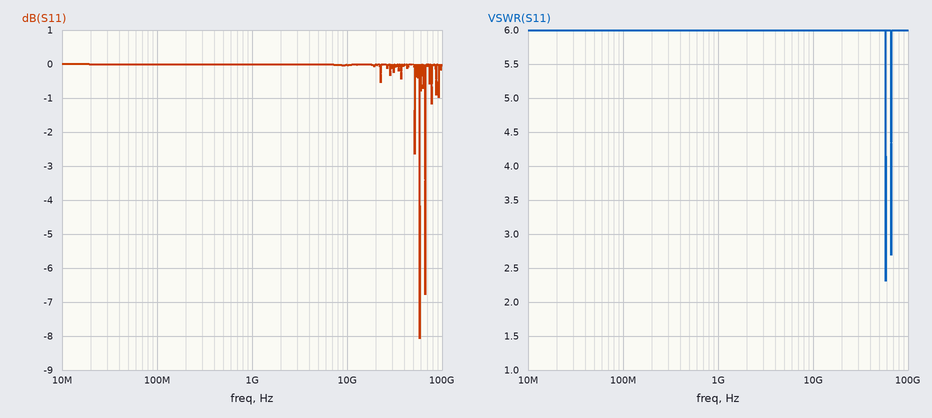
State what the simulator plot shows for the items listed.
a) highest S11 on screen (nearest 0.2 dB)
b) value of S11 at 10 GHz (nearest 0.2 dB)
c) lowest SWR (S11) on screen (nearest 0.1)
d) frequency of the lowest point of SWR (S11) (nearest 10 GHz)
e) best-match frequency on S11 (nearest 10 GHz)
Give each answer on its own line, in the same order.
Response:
0.0 dB
0.0 dB
2.3
60 GHz
60 GHz
